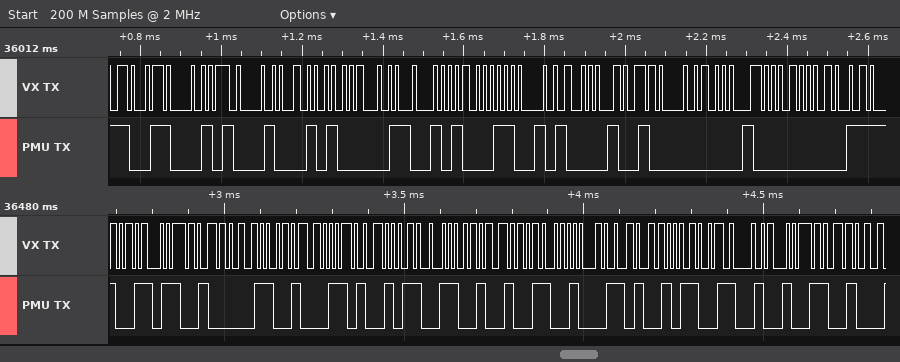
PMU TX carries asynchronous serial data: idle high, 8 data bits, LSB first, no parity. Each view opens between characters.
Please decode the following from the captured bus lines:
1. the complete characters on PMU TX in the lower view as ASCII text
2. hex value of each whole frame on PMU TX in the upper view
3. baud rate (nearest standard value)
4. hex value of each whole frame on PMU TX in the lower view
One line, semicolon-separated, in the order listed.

"60,32,32"; 46, 44, 30, 31, 21, 00, 00; 38400 baud; 36, 30, 2C, 33, 32, 2C, 33, 32
